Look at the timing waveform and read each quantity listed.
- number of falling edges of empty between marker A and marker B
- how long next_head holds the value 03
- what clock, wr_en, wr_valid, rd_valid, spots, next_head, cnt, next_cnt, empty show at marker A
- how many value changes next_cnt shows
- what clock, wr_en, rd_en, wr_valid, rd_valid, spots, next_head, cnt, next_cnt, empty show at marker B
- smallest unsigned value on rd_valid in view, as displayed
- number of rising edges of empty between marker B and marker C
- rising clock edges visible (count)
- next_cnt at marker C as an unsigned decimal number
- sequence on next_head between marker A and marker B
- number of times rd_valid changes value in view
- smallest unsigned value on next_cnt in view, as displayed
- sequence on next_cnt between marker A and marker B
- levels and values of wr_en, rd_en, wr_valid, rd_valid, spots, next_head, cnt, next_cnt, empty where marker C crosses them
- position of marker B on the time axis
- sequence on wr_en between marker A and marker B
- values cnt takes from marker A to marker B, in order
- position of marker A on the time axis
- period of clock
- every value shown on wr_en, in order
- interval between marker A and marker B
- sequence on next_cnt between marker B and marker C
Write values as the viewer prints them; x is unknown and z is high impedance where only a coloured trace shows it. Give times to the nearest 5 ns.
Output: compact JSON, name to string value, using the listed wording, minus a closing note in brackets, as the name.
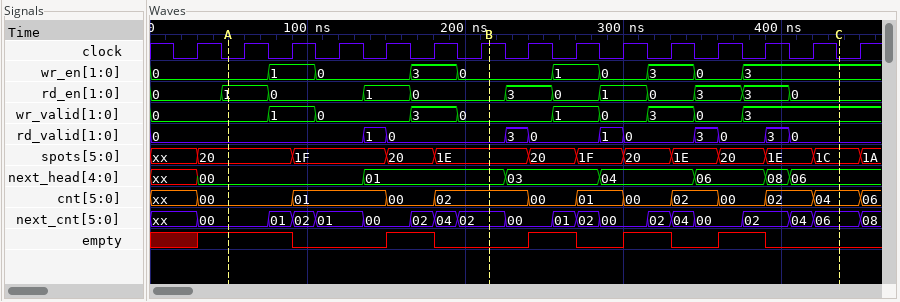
{"number of falling edges of empty between marker A and marker B": "2", "how long next_head holds the value 03": "60 ns", "what clock, wr_en, wr_valid, rd_valid, spots, next_head, cnt, next_cnt, empty show at marker A": "clock=0, wr_en=0, wr_valid=0, rd_valid=0, spots=20, next_head=00, cnt=00, next_cnt=00, empty=1", "how many value changes next_cnt shows": "19", "what clock, wr_en, rd_en, wr_valid, rd_valid, spots, next_head, cnt, next_cnt, empty show at marker B": "clock=1, wr_en=0, rd_en=0, wr_valid=0, rd_valid=0, spots=1E, next_head=01, cnt=02, next_cnt=02, empty=0", "smallest unsigned value on rd_valid in view, as displayed": "0", "number of rising edges of empty between marker B and marker C": "3", "rising clock edges visible": "15", "next_cnt at marker C as an unsigned decimal number": "6", "sequence on next_head between marker A and marker B": "00, 01", "number of times rd_valid changes value in view": "10", "smallest unsigned value on next_cnt in view, as displayed": "00", "sequence on next_cnt between marker A and marker B": "00, 01, 02, 01, 00, 02, 04, 02", "levels and values of wr_en, rd_en, wr_valid, rd_valid, spots, next_head, cnt, next_cnt, empty where marker C crosses them": "wr_en=3, rd_en=0, wr_valid=3, rd_valid=0, spots=1C, next_head=06, cnt=04, next_cnt=06, empty=0", "position of marker B on the time axis": "215 ns", "sequence on wr_en between marker A and marker B": "0, 1, 0, 3, 0", "values cnt takes from marker A to marker B, in order": "00, 01, 00, 02", "position of marker A on the time axis": "50 ns", "period of clock": "30 ns", "every value shown on wr_en, in order": "0, 1, 0, 3, 0, 1, 0, 3, 0, 3", "interval between marker A and marker B": "165 ns", "sequence on next_cnt between marker B and marker C": "02, 00, 01, 02, 00, 02, 04, 00, 02, 04, 06"}
